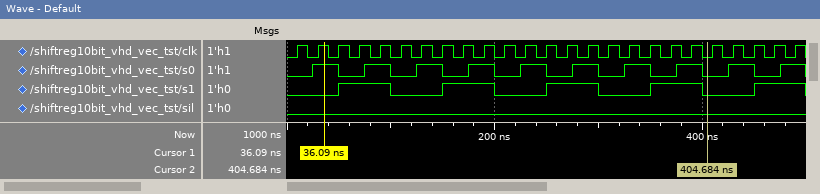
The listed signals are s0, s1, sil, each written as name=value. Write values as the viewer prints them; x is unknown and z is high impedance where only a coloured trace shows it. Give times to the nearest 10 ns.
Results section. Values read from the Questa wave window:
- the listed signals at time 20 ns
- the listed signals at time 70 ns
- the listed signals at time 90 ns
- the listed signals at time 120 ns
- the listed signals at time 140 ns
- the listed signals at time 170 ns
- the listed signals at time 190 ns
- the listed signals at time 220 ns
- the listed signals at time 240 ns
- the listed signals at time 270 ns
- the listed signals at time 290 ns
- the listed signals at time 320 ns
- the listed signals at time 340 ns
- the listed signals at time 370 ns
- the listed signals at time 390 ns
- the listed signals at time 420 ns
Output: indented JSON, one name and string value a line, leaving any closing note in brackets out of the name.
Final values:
{
  "the listed signals at time 20 ns": "s0=0, s1=0, sil=0",
  "the listed signals at time 70 ns": "s0=0, s1=1, sil=0",
  "the listed signals at time 90 ns": "s0=1, s1=1, sil=0",
  "the listed signals at time 120 ns": "s0=0, s1=0, sil=0",
  "the listed signals at time 140 ns": "s0=1, s1=0, sil=0",
  "the listed signals at time 170 ns": "s0=0, s1=1, sil=0",
  "the listed signals at time 190 ns": "s0=1, s1=1, sil=0",
  "the listed signals at time 220 ns": "s0=0, s1=0, sil=0",
  "the listed signals at time 240 ns": "s0=1, s1=0, sil=0",
  "the listed signals at time 270 ns": "s0=0, s1=1, sil=0",
  "the listed signals at time 290 ns": "s0=1, s1=1, sil=0",
  "the listed signals at time 320 ns": "s0=0, s1=0, sil=0",
  "the listed signals at time 340 ns": "s0=1, s1=0, sil=0",
  "the listed signals at time 370 ns": "s0=0, s1=1, sil=0",
  "the listed signals at time 390 ns": "s0=1, s1=1, sil=0",
  "the listed signals at time 420 ns": "s0=0, s1=0, sil=0"
}
